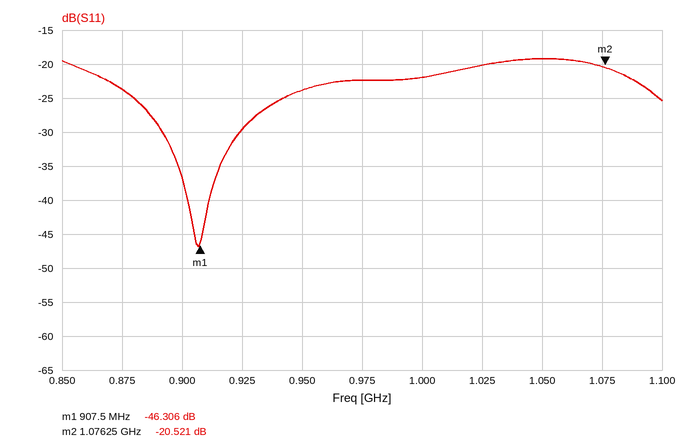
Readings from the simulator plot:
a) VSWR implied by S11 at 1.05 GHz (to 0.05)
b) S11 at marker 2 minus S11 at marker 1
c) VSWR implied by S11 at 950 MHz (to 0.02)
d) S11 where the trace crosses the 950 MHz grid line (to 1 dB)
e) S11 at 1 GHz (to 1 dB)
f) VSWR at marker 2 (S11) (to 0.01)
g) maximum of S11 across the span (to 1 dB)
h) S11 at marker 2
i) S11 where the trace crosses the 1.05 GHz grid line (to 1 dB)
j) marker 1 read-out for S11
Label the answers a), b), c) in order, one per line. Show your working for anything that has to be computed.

a) |Γ| = 10^(-19/20) = 0.1122; VSWR = (1 + 0.1122)/(1 − 0.1122) ≈ 1.25
b) -20.521 − (-46.306) = 25.785 dB
c) |Γ| = 10^(-24/20) = 0.0631; VSWR = (1 + 0.0631)/(1 − 0.0631) ≈ 1.13, so 1.14 to the nearest 0.02
d) -24 dB
e) -22 dB
f) (1 + 0.0942)/(1 − 0.0942) ≈ 1.21
g) -19 dB
h) -20.521 dB
i) -19 dB
j) -46.306 dB
